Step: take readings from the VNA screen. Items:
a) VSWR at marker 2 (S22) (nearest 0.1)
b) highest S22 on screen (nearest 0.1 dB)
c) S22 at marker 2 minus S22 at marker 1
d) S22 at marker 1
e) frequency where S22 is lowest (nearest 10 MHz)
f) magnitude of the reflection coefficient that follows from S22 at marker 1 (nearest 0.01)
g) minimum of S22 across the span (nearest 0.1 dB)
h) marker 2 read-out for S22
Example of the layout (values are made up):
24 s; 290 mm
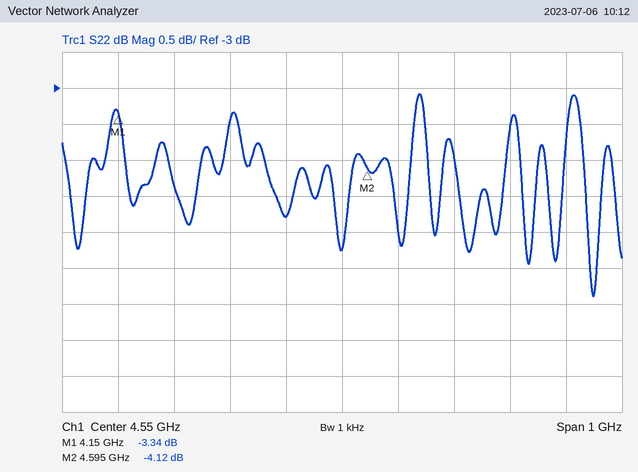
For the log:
4.3; -3.1 dB; -0.78 dB; -3.34 dB; 5.00 GHz; 0.68; -5.9 dB; -4.12 dB
